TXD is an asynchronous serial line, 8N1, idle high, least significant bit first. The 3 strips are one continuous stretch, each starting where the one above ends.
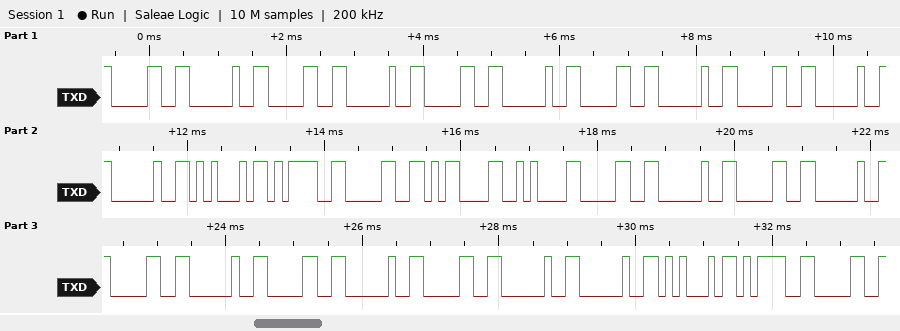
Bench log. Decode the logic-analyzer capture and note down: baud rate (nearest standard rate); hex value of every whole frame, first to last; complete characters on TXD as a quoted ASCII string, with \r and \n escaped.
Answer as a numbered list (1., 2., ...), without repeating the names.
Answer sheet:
1. 9600 baud
2. 30 20 30 20 30 20 30 20 30 20 20 45 3D 30 0D 0A 30 20 30 20 30 20 30 20 30 20 20 45 3D 30
3. "0 0 0 0 0  E=0\r\n0 0 0 0 0  E=0"
